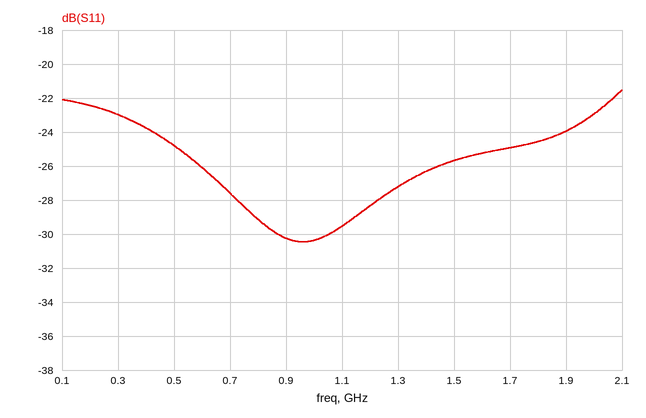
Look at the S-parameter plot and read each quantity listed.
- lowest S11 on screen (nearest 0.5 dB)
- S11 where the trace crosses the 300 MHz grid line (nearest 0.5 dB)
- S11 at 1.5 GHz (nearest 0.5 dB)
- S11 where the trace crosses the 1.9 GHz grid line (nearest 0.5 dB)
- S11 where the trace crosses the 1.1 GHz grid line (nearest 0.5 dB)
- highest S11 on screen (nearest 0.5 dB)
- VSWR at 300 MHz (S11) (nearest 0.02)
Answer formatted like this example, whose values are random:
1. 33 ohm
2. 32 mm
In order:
1. -30.5 dB
2. -23.0 dB
3. -25.5 dB
4. -24.0 dB
5. -29.5 dB
6. -21.5 dB
7. 1.16
